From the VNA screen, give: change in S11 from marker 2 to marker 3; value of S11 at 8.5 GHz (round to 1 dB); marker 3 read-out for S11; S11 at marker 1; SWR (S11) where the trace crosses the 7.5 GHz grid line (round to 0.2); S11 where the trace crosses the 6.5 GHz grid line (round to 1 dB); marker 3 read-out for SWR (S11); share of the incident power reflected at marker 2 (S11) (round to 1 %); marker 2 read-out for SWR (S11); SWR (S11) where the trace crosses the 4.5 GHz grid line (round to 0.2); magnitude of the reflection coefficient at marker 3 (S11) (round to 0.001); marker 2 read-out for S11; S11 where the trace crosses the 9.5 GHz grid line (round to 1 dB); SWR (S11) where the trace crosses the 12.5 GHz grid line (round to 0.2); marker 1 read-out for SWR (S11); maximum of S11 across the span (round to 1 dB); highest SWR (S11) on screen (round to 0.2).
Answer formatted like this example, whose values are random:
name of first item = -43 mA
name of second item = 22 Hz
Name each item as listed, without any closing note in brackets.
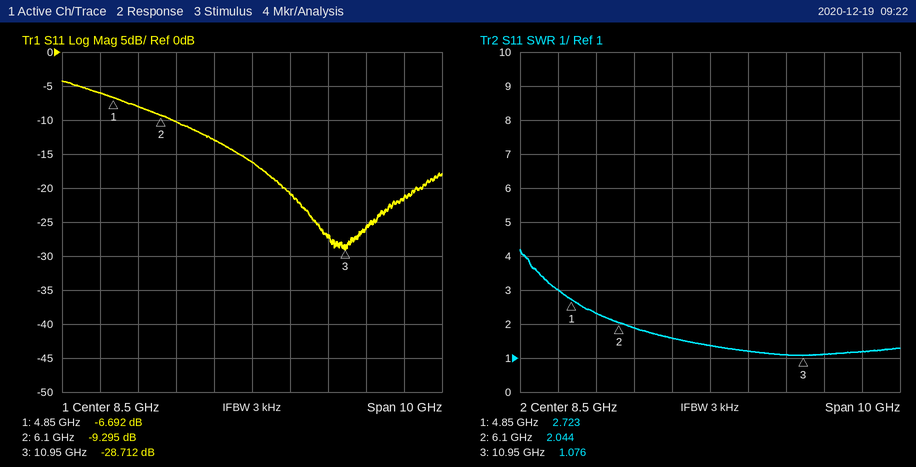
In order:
change in S11 from marker 2 to marker 3 = -19.417 dB
value of S11 at 8.5 GHz = -16 dB
marker 3 read-out for S11 = -28.712 dB
S11 at marker 1 = -6.692 dB
SWR (S11) where the trace crosses the 7.5 GHz grid line = 1.6
S11 where the trace crosses the 6.5 GHz grid line = -10 dB
marker 3 read-out for SWR = 1.076
share of the incident power reflected at marker 2 (S11) = 12 %
marker 2 read-out for SWR = 2.044
SWR (S11) where the trace crosses the 4.5 GHz grid line = 3.0
magnitude of the reflection coefficient at marker 3 (S11) = 0.037
marker 2 read-out for S11 = -9.295 dB
S11 where the trace crosses the 9.5 GHz grid line = -21 dB
SWR (S11) where the trace crosses the 12.5 GHz grid line = 1.2
marker 1 read-out for SWR = 2.723
maximum of S11 across the span = -4 dB
highest SWR (S11) on screen = 4.2
